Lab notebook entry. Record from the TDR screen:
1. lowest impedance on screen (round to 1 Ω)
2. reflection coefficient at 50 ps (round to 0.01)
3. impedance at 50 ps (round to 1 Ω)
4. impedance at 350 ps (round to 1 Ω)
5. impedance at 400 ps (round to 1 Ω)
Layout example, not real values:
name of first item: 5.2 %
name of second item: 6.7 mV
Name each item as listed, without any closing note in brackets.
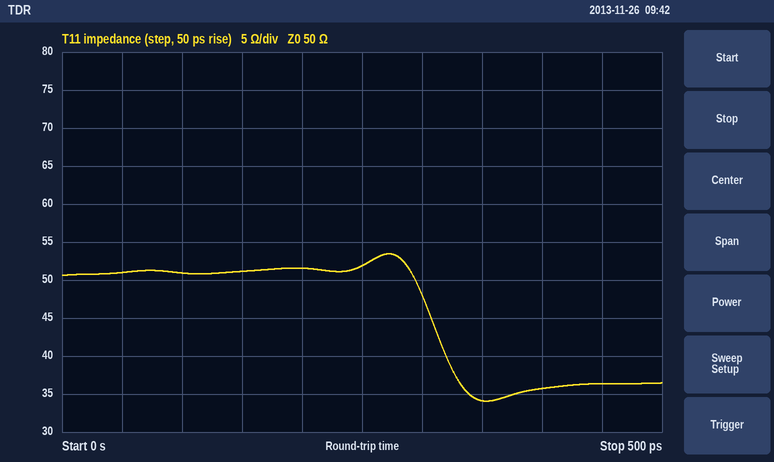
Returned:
lowest impedance on screen: 34 Ω
reflection coefficient at 50 ps: +0.01
impedance at 50 ps: 51 Ω
impedance at 350 ps: 34 Ω
impedance at 400 ps: 36 Ω
